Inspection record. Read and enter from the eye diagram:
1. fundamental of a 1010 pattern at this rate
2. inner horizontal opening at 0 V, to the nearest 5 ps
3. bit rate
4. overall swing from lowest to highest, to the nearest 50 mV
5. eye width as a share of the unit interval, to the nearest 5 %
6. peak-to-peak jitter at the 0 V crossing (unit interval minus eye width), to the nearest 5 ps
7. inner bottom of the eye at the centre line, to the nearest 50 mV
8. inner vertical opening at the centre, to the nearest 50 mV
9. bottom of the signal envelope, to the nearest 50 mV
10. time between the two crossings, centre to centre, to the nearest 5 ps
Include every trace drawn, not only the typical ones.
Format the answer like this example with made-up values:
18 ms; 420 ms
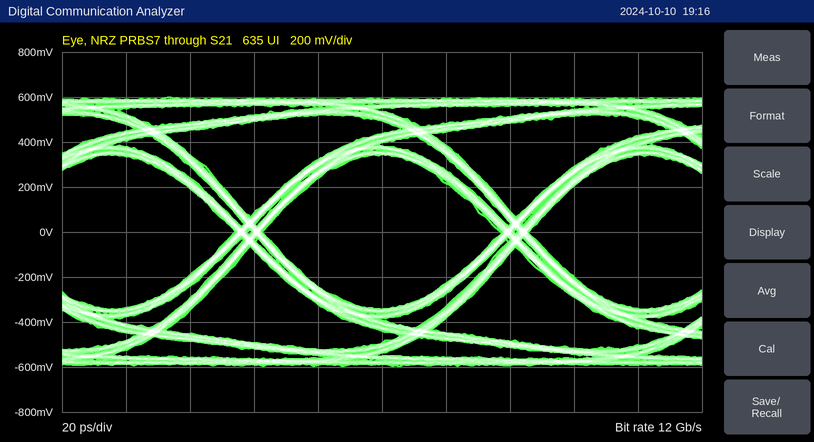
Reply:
6 GHz; 75 ps; 12 Gb/s; 1.20 V; 90 %; 10 ps; -350 mV; 700 mV; -600 mV; 85 ps
